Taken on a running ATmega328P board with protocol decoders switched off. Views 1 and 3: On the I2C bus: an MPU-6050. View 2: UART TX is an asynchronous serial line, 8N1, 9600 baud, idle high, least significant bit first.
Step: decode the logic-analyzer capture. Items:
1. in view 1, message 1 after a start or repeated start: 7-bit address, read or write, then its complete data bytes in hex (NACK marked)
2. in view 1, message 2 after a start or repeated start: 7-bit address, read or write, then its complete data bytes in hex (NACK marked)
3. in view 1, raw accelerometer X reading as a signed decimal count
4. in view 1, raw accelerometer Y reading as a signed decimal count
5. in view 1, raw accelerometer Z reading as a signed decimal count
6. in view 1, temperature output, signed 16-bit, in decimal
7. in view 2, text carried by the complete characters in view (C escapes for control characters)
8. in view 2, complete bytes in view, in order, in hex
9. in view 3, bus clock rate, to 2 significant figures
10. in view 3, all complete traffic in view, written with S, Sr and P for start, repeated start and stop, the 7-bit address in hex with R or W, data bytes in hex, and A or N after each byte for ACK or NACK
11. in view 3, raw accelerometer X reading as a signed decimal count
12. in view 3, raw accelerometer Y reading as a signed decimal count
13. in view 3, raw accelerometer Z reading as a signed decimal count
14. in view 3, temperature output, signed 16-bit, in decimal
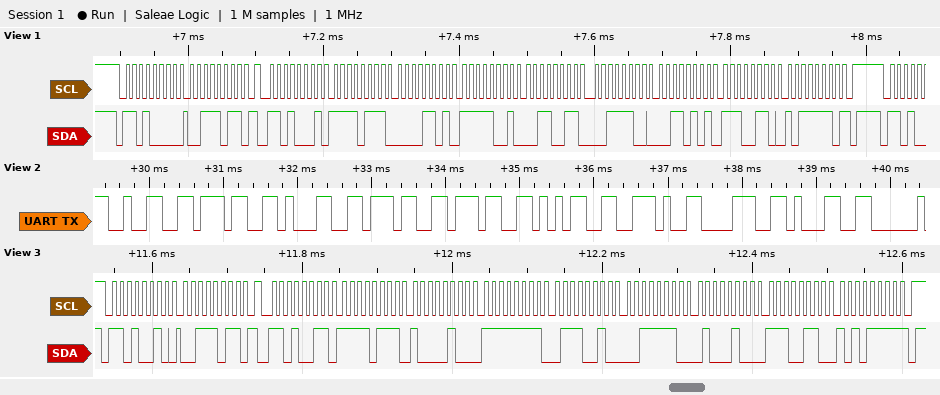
0x68 write: 3B
0x68 read: F7 0D F9 33 3C 35 E6 BE NACK
-2291
-1741
15413
-6466
"271775.81"
32 37 31 37 37 35 2E 38 31
100 kHz
S 69W A 3B A Sr 69R A F7 A 84 A FF A 72 A 3E A 44 A E6 A AF N P
-2172
-142
15940
-6481
